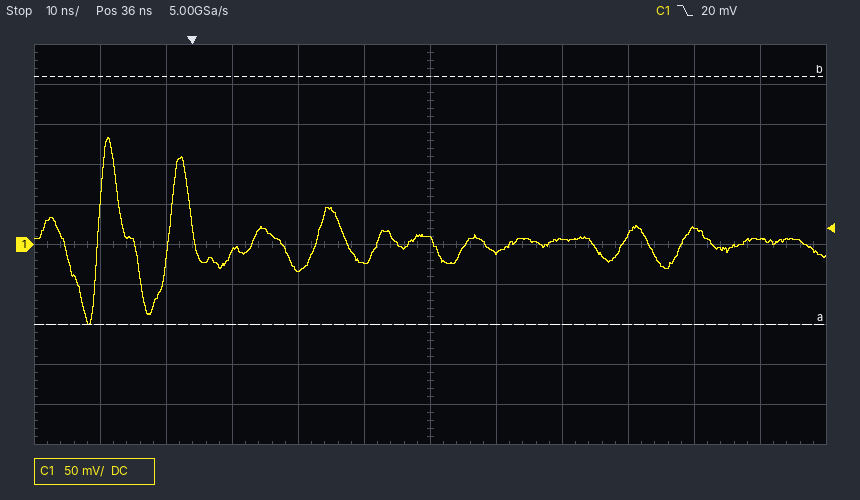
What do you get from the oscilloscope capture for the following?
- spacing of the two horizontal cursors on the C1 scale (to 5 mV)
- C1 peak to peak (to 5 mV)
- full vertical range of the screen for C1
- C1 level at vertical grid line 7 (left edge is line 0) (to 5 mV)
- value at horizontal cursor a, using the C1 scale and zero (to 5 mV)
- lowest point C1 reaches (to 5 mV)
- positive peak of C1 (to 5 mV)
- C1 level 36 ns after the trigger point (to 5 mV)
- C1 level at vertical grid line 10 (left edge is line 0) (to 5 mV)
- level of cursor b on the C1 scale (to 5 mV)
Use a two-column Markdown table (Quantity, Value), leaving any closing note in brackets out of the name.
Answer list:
| Quantity | Value |
|---|---|
| spacing of the two horizontal cursors on the C1 scale | 310 mV |
| C1 peak to peak | 235 mV |
| full vertical range of the screen for C1 | 500 mV |
| C1 level at vertical grid line 7 (left edge is line 0) | -10 mV |
| value at horizontal cursor a, using the C1 scale and zero | -100 mV |
| lowest point C1 reaches | -100 mV |
| positive peak of C1 | 135 mV |
| C1 level 36 ns after the trigger point | 5 mV |
| C1 level at vertical grid line 10 (left edge is line 0) | 20 mV |
| level of cursor b on the C1 scale | 210 mV |
